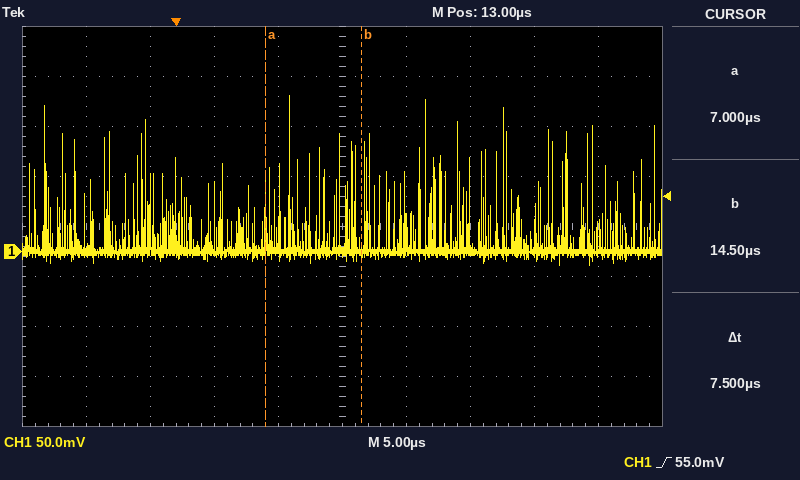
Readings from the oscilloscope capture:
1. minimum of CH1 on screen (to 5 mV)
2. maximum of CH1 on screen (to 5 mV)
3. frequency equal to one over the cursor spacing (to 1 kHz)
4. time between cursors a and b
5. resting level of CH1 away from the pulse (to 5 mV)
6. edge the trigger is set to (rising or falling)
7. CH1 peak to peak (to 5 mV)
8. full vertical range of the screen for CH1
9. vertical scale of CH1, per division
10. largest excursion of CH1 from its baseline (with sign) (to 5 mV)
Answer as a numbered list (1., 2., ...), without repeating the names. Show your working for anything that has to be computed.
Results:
1. -15 mV
2. 155 mV
3. 1 / 7.5 µs ≈ 133 kHz
4. 7.5 µs
5. 0 mV
6. rising
7. 155 mV − (-15 mV) = 170 mV
8. 400 mV
9. 50 mV
10. 155 mV − (0 mV) = +155 mV
